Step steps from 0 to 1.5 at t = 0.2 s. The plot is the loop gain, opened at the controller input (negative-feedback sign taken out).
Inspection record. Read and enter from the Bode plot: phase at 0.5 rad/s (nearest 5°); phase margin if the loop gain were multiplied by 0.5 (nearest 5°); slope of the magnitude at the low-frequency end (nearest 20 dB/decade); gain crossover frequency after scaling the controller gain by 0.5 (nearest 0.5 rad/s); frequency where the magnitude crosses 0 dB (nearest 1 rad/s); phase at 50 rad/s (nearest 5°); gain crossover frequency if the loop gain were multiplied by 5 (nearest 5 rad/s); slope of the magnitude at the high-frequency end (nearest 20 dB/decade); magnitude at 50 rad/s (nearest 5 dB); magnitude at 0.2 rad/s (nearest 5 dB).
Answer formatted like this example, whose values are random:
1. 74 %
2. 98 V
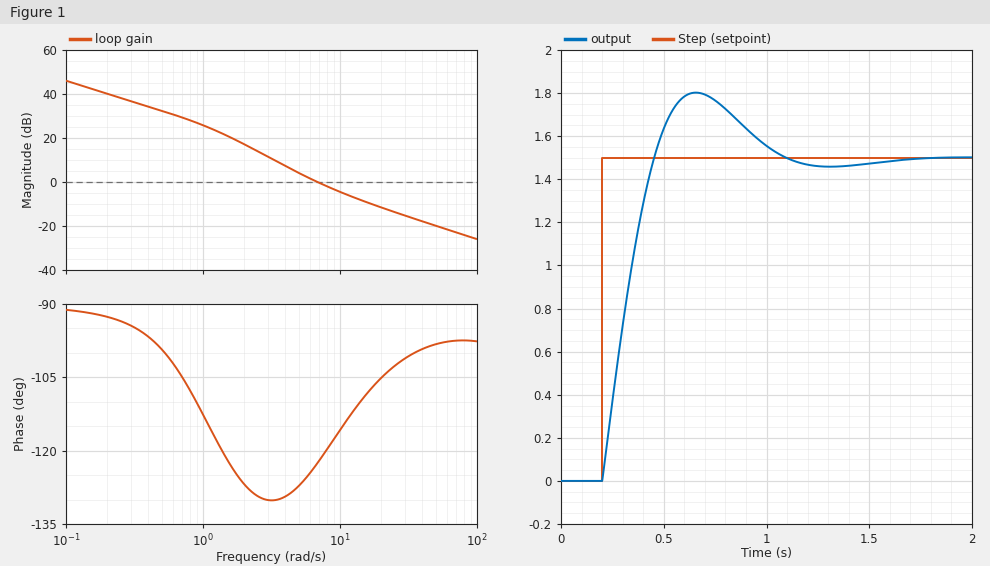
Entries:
1. -100°
2. 50°
3. -20 dB/decade
4. 4.5 rad/s
5. 7 rad/s
6. -100°
7. 25 rad/s
8. -20 dB/decade
9. -20 dB
10. 40 dB
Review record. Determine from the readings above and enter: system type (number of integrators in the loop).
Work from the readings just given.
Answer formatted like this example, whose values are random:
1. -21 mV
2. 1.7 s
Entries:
1. 1
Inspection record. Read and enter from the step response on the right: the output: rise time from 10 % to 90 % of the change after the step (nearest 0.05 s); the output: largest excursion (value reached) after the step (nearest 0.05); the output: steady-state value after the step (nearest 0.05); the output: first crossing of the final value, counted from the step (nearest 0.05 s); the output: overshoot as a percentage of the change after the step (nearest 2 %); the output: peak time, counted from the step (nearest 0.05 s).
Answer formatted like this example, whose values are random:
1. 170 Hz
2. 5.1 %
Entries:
1. 0.20 s
2. 1.80
3. 1.50
4. 0.25 s
5. 20 %
6. 0.45 s
